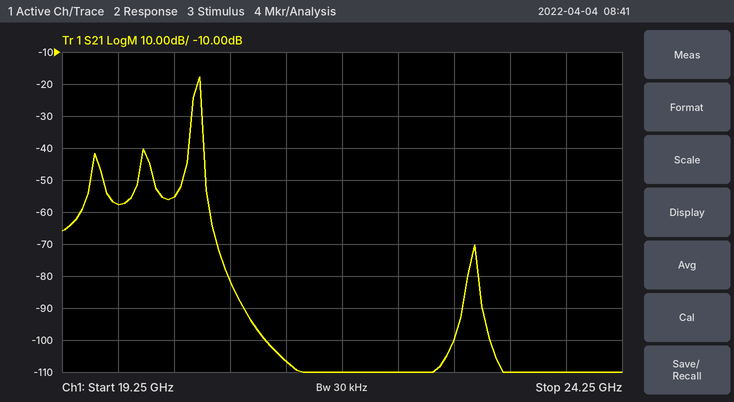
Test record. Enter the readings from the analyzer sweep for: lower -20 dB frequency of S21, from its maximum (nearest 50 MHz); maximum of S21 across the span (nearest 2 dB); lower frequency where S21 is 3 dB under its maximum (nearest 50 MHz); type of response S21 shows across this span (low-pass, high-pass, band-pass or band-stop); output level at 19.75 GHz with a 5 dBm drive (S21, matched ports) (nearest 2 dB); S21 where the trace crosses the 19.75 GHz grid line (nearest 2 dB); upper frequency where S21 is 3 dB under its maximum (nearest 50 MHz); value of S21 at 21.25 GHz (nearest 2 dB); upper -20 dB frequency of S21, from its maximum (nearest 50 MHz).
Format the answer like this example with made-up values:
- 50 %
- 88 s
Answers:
- 20.40 GHz
- -18 dB
- 20.45 GHz
- band-pass
- -52 dBm
- -58 dB
- 20.50 GHz
- -106 dB
- 20.50 GHz
